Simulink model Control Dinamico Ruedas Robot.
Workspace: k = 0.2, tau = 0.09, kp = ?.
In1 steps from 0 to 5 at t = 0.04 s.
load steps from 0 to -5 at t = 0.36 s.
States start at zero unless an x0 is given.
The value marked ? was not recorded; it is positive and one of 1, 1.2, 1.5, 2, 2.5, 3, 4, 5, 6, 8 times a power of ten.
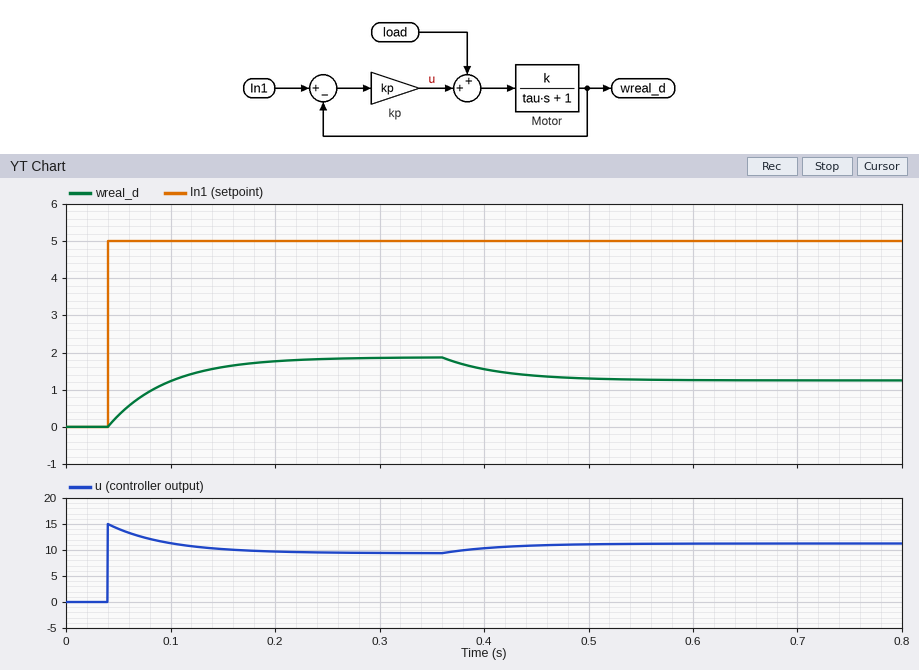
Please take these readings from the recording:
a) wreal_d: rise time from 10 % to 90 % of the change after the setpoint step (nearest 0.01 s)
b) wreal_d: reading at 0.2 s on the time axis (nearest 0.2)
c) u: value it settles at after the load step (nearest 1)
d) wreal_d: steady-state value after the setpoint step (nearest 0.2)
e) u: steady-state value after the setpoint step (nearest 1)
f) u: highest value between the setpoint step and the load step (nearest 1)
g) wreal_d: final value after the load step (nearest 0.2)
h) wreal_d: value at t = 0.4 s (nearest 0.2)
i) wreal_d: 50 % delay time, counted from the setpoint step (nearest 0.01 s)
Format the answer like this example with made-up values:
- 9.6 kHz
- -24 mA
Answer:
- 0.12 s
- 1.8
- 11
- 1.8
- 9
- 15
- 1.2
- 1.6
- 0.04 s
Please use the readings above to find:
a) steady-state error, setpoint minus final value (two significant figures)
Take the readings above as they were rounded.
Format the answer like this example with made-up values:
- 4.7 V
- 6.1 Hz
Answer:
- 3.2
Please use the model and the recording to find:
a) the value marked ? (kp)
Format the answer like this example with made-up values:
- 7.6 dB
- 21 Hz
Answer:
- 3
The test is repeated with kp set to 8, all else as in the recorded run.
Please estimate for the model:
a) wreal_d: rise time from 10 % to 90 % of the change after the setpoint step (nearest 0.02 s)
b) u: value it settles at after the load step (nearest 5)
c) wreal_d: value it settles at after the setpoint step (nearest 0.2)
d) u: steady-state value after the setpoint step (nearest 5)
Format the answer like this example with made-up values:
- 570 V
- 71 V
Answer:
- 0.08 s
- 20
- 3.0
- 15
